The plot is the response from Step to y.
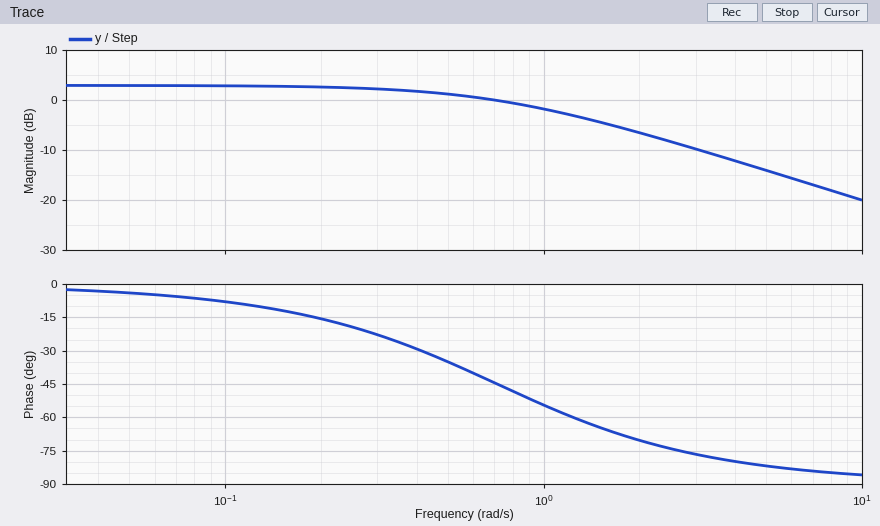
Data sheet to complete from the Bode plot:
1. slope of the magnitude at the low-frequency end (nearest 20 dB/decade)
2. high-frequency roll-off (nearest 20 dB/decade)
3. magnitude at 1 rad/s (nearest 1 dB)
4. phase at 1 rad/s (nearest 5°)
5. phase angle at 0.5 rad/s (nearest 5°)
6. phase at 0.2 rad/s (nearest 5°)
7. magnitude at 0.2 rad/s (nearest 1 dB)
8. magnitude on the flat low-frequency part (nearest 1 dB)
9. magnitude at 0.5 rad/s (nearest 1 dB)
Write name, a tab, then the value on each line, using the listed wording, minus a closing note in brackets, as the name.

slope of the magnitude at the low-frequency end	0 dB/decade
high-frequency roll-off	-20 dB/decade
magnitude at 1 rad/s	-2 dB
phase at 1 rad/s	-55°
phase angle at 0.5 rad/s	-35°
phase at 0.2 rad/s	-15°
magnitude at 0.2 rad/s	3 dB
magnitude on the flat low-frequency part	3 dB
magnitude at 0.5 rad/s	1 dB
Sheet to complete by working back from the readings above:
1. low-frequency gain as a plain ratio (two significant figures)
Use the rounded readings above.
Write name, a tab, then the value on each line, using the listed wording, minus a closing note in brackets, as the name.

low-frequency gain as a plain ratio	1.4
